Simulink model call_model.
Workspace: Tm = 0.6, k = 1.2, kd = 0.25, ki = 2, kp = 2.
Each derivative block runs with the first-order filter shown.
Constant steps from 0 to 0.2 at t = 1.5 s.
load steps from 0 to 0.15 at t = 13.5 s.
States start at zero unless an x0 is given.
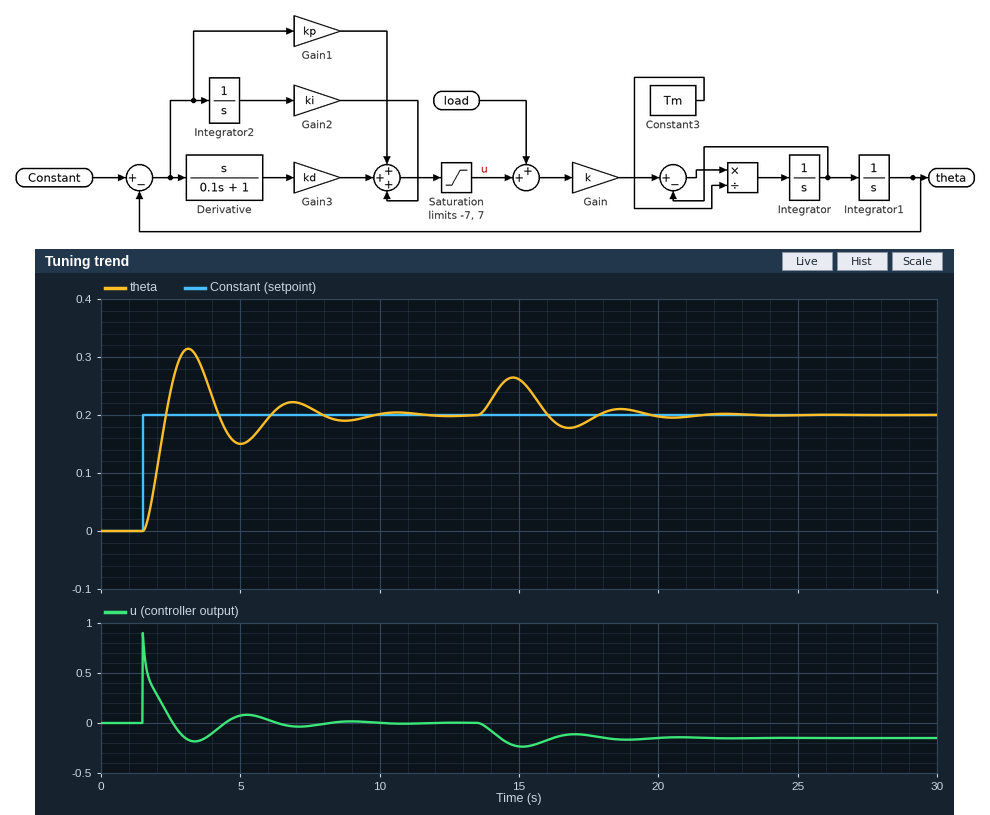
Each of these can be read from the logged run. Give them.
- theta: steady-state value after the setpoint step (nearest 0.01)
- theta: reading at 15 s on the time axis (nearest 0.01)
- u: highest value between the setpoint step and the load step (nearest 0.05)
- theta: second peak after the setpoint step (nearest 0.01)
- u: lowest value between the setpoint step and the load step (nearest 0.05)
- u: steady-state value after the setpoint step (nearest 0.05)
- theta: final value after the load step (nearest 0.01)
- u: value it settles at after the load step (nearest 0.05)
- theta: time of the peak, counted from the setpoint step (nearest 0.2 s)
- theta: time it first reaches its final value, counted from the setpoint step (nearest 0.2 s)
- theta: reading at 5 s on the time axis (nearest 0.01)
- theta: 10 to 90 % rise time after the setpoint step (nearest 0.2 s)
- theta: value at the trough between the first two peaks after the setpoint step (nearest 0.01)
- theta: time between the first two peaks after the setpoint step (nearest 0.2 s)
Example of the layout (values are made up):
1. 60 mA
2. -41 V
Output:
1. 0.20
2. 0.26
3. 0.90
4. 0.22
5. -0.20
6. 0.00
7. 0.20
8. -0.15
9. 1.6 s
10. 0.8 s
11. 0.15
12. 0.6 s
13. 0.15
14. 3.8 s
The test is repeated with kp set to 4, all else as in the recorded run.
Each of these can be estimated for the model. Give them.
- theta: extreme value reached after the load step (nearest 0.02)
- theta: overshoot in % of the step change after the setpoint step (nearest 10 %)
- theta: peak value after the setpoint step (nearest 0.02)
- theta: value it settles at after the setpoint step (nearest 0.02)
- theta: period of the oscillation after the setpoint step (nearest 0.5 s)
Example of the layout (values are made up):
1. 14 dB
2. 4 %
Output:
1. 0.24
2. 50 %
3. 0.30
4. 0.20
5. 2.5 s
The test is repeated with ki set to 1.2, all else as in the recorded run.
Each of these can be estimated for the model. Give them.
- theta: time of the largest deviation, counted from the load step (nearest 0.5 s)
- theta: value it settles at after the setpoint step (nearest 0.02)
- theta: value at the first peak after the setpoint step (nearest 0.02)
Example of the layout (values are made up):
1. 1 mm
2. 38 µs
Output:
1. 1.5 s
2. 0.20
3. 0.28
